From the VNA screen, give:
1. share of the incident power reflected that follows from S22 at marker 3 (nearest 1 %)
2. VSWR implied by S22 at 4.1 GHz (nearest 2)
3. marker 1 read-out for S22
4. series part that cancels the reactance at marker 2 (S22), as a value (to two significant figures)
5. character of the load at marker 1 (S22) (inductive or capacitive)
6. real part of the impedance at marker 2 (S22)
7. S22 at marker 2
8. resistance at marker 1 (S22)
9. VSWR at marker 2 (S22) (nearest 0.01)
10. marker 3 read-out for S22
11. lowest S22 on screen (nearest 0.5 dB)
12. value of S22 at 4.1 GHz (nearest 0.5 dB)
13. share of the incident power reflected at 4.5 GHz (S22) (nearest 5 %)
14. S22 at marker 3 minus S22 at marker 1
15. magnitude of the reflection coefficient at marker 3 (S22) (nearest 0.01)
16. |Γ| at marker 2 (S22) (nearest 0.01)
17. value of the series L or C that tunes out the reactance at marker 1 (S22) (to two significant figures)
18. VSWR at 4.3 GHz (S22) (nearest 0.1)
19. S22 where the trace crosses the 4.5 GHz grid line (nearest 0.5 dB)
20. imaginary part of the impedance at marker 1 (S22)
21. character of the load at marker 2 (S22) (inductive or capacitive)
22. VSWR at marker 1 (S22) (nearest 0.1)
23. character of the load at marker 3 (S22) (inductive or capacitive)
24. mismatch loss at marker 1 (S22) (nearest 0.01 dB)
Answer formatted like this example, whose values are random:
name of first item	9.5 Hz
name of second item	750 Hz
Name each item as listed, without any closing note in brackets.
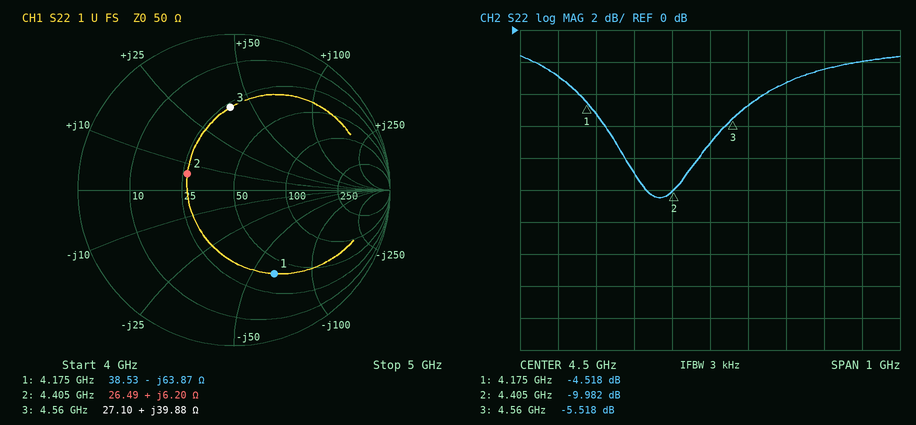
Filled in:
share of the incident power reflected that follows from S22 at marker 3	28 %
VSWR implied by S22 at 4.1 GHz	6
marker 1 read-out for S22	-4.518 dB
series part that cancels the reactance at marker 2 (S22), as a value	5.8 pF
character of the load at marker 1 (S22)	capacitive
real part of the impedance at marker 2	26.49 Ω
S22 at marker 2	-9.982 dB
resistance at marker 1	38.53 Ω
VSWR at marker 2 (S22)	1.93
marker 3 read-out for S22	-5.518 dB
lowest S22 on screen	-10.5 dB
value of S22 at 4.1 GHz	-3.0 dB
share of the incident power reflected at 4.5 GHz (S22)	20 %
S22 at marker 3 minus S22 at marker 1	-1.000 dB
magnitude of the reflection coefficient at marker 3 (S22)	0.53
|Γ| at marker 2 (S22)	0.32
value of the series L or C that tunes out the reactance at marker 1 (S22)	2.4 nH
VSWR at 4.3 GHz (S22)	2.1
S22 where the trace crosses the 4.5 GHz grid line	-7.0 dB
imaginary part of the impedance at marker 1	-63.87 Ω
character of the load at marker 2 (S22)	inductive
VSWR at marker 1 (S22)	3.9
character of the load at marker 3 (S22)	inductive
mismatch loss at marker 1 (S22)	1.89 dB
